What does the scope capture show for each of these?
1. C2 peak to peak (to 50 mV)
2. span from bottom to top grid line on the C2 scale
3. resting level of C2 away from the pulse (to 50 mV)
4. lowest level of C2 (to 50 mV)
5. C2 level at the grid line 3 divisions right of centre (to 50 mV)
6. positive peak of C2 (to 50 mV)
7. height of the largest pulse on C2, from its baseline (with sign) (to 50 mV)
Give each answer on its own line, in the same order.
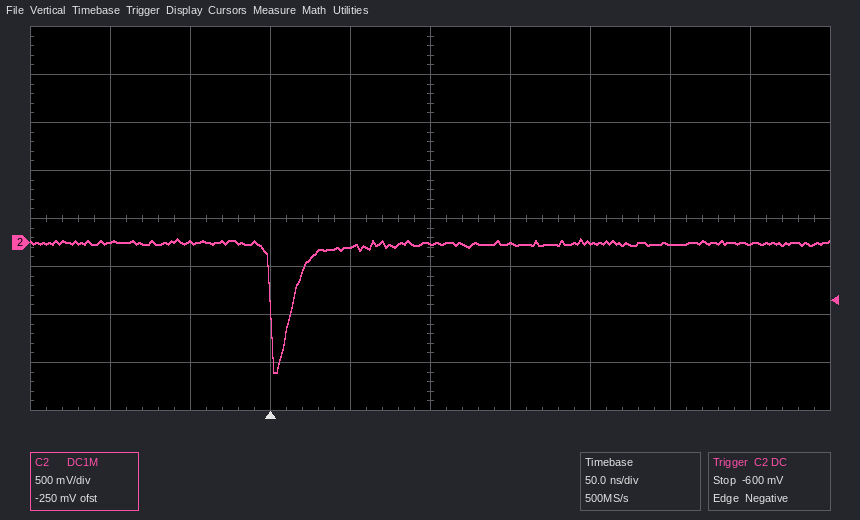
1.40 V
4 V
0 mV
-1.35 V
0 mV
50 mV
-1.35 V
